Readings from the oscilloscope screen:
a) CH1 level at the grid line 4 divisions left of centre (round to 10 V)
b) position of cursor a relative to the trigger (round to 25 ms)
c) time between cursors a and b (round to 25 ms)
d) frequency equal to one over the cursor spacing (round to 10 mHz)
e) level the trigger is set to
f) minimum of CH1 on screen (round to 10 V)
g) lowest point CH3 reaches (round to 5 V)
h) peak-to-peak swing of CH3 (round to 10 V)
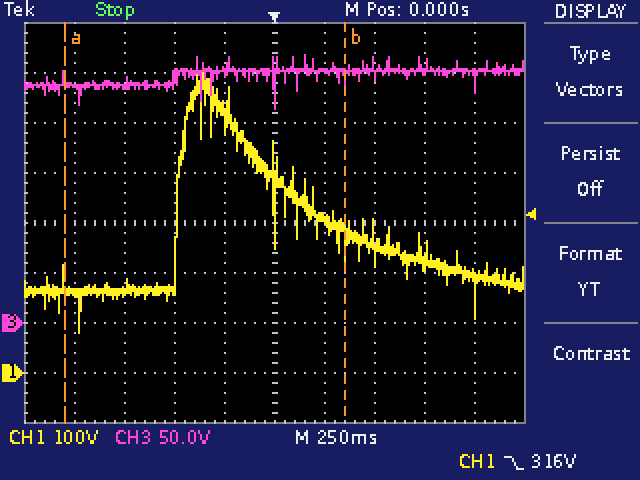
160 V
-1.050 s
1.400 s
710 mHz
316 V
80 V
215 V
50 V
